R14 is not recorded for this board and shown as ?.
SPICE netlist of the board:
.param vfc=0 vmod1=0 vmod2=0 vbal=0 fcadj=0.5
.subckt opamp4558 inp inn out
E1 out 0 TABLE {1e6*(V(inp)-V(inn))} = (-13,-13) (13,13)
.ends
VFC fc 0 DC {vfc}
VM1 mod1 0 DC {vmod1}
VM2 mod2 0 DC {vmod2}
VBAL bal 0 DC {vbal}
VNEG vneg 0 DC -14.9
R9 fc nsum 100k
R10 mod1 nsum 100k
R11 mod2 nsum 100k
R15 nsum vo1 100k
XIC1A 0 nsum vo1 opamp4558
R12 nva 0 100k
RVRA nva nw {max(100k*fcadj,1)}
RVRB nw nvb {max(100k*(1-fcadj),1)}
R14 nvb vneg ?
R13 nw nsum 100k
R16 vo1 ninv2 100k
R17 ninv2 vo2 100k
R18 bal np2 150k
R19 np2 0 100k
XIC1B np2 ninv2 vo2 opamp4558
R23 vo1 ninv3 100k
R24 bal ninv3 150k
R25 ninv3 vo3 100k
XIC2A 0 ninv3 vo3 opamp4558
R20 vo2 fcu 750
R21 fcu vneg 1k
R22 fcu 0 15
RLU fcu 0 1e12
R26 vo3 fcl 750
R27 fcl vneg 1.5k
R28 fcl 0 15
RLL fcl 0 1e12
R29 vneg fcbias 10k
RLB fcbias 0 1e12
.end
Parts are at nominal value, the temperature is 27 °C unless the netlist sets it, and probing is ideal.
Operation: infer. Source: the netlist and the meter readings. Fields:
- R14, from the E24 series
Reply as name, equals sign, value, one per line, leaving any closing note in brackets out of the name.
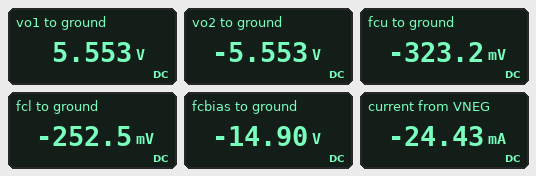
R14, from the E24 series = 51 kΩ
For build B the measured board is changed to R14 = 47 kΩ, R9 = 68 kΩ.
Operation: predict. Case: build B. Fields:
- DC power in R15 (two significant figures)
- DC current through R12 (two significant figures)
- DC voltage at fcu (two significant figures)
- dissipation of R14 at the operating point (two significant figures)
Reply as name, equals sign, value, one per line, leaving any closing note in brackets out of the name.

DC power in R15 = 320 µW
DC current through R12 = 38 µA
DC voltage at fcu = -330 mV
dissipation of R14 at the operating point = 420 µW
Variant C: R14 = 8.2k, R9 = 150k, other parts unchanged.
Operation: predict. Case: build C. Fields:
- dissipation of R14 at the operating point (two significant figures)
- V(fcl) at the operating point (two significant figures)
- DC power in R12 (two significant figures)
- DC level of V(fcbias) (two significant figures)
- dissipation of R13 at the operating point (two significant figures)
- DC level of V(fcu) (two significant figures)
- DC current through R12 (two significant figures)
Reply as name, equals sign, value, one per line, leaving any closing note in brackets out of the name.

dissipation of R14 at the operating point = 130 µW
V(fcl) at the operating point = -290 mV
DC power in R12 = 250 µW
DC level of V(fcbias) = -15 V
dissipation of R13 at the operating point = 570 µW
DC level of V(fcu) = -360 mV
DC current through R12 = 50 µA
